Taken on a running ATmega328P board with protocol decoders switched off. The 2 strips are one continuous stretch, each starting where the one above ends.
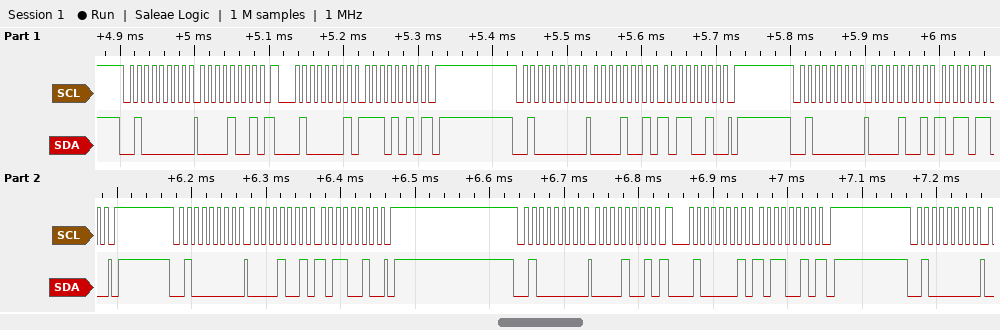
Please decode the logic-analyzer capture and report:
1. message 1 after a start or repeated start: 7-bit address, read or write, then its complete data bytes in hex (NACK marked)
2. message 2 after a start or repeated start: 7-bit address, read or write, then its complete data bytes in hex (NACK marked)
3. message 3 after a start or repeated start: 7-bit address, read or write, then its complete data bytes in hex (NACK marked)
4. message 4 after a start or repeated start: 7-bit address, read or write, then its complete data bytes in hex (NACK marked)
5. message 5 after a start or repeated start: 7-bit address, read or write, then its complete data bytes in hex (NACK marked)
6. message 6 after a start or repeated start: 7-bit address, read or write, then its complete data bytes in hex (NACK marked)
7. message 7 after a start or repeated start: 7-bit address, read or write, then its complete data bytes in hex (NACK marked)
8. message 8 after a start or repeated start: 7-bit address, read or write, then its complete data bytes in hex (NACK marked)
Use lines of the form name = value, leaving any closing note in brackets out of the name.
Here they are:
message 1 after a start or repeated start: 7-bit address, read or write, then its complete data bytes in hex = 0x20 write: 09
message 2 after a start or repeated start: 7-bit address, read or write, then its complete data bytes in hex = 0x20 read: EA NACK
message 3 after a start or repeated start: 7-bit address, read or write, then its complete data bytes in hex = 0x20 write: 09 B2
message 4 after a start or repeated start: 7-bit address, read or write, then its complete data bytes in hex = 0x20 write: 09 B6
message 5 after a start or repeated start: 7-bit address, read or write, then its complete data bytes in hex = 0x20 write: 09 B2
message 6 after a start or repeated start: 7-bit address, read or write, then its complete data bytes in hex = 0x20 write: 09
message 7 after a start or repeated start: 7-bit address, read or write, then its complete data bytes in hex = 0x20 read: B2 NACK
message 8 after a start or repeated start: 7-bit address, read or write, then its complete data bytes in hex = 0x20 write
